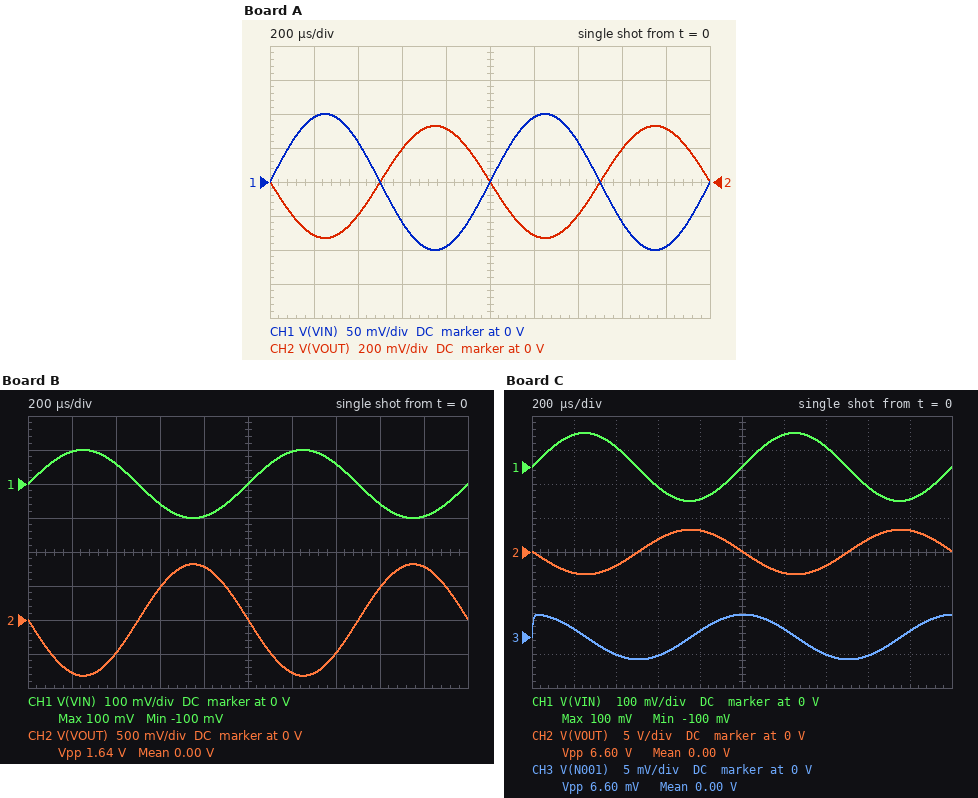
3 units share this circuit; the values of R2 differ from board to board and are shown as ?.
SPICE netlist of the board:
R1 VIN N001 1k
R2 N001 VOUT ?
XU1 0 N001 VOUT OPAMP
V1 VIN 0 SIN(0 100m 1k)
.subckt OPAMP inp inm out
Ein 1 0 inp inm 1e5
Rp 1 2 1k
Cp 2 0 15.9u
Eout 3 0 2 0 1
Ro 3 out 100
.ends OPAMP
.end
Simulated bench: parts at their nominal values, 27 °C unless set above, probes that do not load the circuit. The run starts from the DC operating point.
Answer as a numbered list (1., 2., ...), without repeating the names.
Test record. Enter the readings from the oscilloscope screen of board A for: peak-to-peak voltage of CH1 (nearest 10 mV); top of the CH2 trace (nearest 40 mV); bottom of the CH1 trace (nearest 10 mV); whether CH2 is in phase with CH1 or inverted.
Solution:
1. 200 mV
2. 320 mV
3. -100 mV
4. inverted
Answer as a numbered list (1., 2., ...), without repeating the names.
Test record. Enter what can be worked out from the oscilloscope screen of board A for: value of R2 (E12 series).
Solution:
1. 3.3 kΩ
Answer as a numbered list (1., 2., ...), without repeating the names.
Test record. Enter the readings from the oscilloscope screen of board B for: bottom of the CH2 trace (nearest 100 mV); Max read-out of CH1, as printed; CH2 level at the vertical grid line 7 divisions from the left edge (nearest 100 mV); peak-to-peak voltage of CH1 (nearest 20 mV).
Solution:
1. -800 mV
2. 100 mV
3. -500 mV
4. 200 mV
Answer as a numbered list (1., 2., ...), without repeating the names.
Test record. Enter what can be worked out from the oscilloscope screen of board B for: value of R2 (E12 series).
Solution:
1. 8.2 kΩ
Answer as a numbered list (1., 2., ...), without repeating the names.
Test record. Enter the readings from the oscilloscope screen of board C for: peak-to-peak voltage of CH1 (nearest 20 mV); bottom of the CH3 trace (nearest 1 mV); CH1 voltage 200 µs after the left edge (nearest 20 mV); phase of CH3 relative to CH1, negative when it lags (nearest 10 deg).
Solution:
1. 200 mV
2. -3 mV
3. 100 mV
4. 90 deg
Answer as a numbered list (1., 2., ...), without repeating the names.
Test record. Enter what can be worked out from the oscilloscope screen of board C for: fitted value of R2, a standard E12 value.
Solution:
1. 33 kΩ
